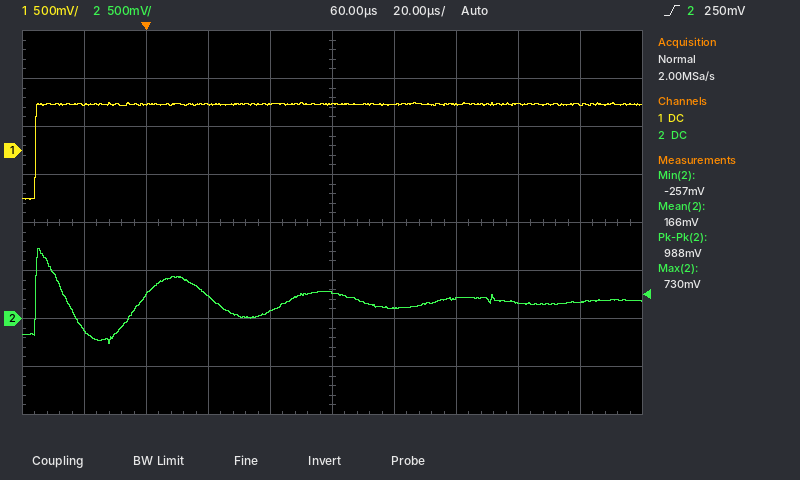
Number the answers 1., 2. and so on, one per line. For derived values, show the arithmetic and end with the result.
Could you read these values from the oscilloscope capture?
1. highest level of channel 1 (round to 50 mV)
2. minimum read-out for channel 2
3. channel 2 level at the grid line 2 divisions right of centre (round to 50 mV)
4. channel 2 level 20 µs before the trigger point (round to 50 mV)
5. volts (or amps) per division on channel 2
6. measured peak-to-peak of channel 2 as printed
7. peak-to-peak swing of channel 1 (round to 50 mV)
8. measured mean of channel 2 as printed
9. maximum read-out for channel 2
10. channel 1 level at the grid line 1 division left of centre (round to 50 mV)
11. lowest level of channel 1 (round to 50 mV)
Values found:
1. 500 mV
2. -257 mV
3. 200 mV
4. -100 mV
5. 500 mV
6. 988 mV
7. 500 mV − (-500 mV) = 1.00 V
8. 166 mV
9. 730 mV
10. 500 mV
11. -500 mV
